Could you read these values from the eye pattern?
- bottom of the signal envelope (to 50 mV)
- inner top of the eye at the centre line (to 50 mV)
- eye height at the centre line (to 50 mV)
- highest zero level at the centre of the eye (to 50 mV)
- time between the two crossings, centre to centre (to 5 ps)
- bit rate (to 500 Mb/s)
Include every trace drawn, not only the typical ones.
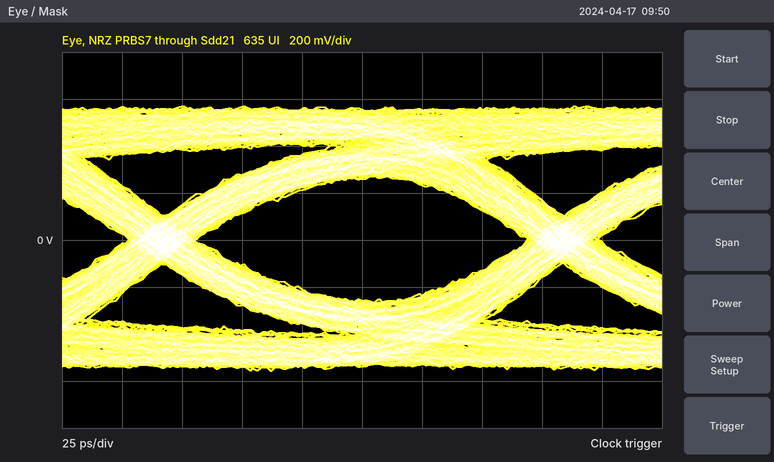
-550 mV
250 mV
500 mV
-250 mV
165 ps
6.0 Gb/s
